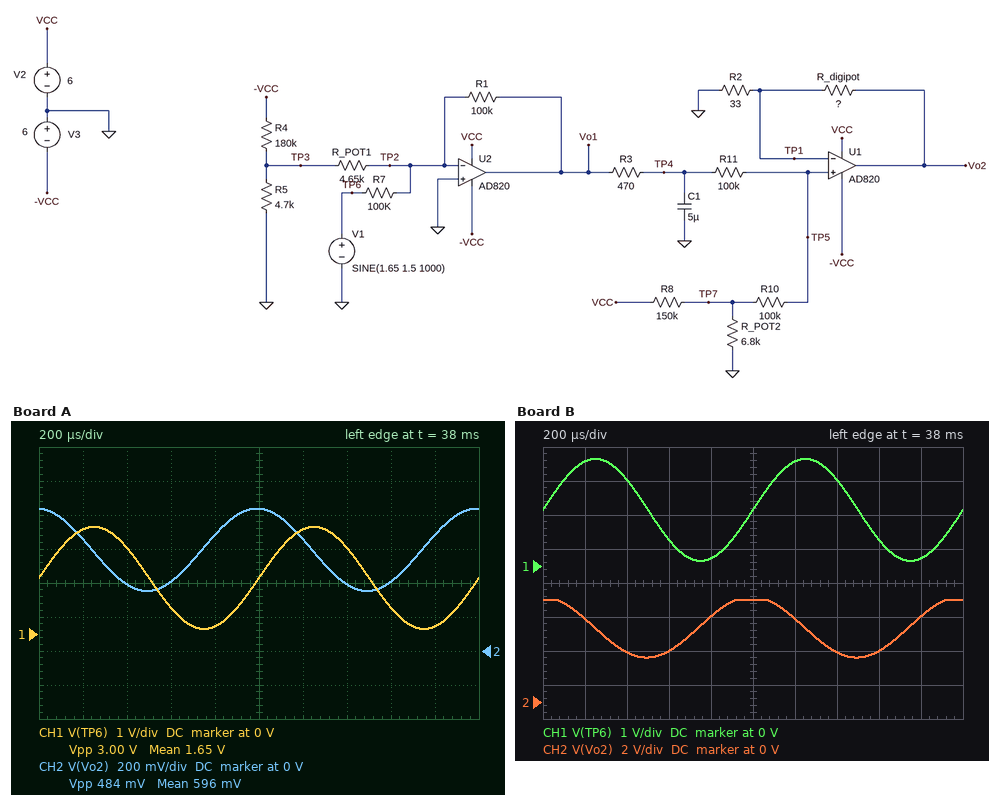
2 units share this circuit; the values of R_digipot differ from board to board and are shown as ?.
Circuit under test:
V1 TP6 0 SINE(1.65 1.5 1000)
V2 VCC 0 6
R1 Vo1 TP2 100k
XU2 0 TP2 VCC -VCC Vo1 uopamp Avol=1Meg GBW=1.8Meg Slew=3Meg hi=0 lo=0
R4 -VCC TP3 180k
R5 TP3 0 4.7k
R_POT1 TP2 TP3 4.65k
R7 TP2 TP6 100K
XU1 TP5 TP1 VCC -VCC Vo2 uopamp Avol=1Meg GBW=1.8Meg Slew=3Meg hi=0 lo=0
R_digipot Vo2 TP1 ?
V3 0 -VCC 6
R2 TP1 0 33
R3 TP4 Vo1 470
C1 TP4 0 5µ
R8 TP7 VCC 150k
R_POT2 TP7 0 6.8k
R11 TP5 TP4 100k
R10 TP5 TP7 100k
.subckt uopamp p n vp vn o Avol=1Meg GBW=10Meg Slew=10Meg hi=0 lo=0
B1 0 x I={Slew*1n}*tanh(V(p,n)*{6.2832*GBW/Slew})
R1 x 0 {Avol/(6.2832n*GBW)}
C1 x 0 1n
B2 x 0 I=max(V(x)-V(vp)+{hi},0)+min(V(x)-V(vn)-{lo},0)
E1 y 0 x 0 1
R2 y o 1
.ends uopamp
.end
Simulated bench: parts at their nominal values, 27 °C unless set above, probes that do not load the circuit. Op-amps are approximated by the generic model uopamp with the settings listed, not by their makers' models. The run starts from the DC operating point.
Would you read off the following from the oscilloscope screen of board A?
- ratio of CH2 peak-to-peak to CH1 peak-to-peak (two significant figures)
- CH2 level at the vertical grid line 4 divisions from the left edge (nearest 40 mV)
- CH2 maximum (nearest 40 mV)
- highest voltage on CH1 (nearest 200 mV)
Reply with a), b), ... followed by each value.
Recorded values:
a) 0.16
b) 680 mV
c) 840 mV
d) 3.2 V
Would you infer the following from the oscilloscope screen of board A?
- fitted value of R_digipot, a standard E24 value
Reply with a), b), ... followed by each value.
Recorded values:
a) 120 Ω
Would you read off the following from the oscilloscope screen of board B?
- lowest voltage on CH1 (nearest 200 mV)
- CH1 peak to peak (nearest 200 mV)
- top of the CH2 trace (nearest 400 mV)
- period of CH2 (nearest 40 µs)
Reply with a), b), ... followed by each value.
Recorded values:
a) 200 mV
b) 3.0 V
c) 6.0 V
d) 1.00 ms
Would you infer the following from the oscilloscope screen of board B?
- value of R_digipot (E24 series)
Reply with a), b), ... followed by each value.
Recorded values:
a) 1.1 kΩ
